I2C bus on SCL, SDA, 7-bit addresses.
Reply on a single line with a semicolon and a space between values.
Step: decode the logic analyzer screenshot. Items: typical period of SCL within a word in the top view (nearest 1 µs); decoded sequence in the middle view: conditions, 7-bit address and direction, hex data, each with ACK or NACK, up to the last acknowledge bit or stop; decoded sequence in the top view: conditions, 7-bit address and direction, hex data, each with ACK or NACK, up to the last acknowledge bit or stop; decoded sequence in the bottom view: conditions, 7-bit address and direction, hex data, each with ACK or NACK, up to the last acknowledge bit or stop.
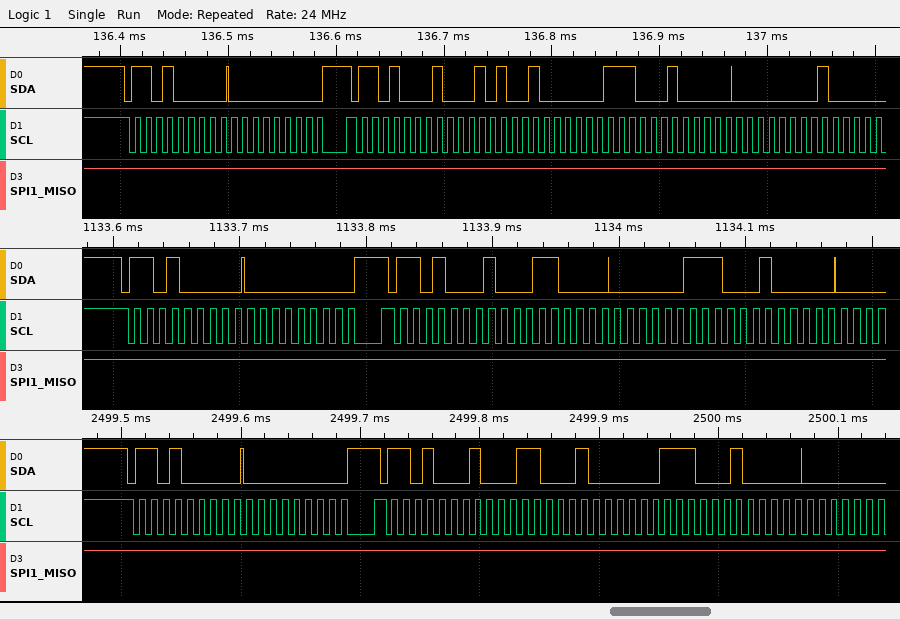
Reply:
10 µs; start, address 68 write ACK, 00 ACK, repeated start, address 68 read ACK, 30 ACK, 07 ACK, 20 ACK; start, address 68 write ACK, 00 ACK, repeated start, address 68 read ACK, 29 ACK, 07 ACK, 20 ACK, 01 ACK; start, address 68 write ACK, 00 ACK, repeated start, address 68 read ACK, 31 ACK, 07 ACK, 20 ACK
